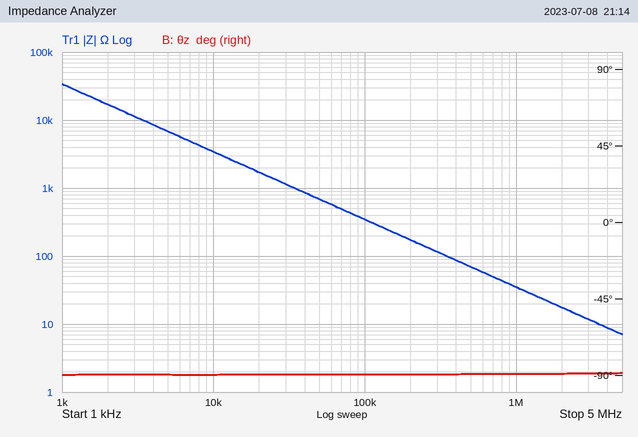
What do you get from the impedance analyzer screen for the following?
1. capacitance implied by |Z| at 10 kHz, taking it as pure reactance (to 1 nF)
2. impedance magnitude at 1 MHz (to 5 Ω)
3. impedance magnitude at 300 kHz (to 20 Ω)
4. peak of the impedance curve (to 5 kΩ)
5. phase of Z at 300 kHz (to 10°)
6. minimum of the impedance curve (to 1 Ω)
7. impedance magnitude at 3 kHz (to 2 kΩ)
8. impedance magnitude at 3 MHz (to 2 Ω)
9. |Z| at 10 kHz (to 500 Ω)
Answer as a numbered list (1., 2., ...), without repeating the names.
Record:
1. 5 nF
2. 35 Ω
3. 120 Ω
4. 35 kΩ
5. -90°
6. 7 Ω
7. 12 kΩ
8. 12 Ω
9. 3.5 kΩ
